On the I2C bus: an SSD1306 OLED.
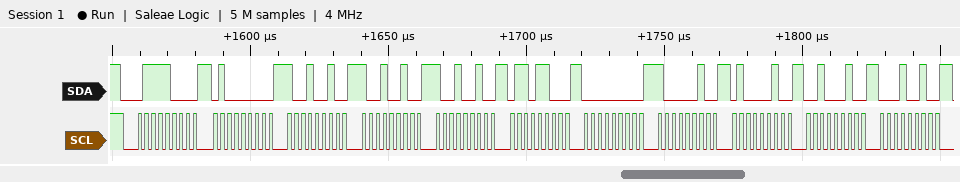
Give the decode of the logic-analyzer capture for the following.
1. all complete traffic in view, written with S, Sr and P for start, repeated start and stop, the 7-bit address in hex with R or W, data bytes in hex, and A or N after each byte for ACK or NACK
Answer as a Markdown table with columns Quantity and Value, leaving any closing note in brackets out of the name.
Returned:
| Quantity | Value |
|---|---|
| all complete traffic in view, written with S, Sr and P for start, repeated start and stop, the 7-bit address in hex with R or W, data bytes in hex, and A or N after each byte for ACK or NACK | S 3CW A 40 A 92 A 92 A 92 A 6C A 00 A 82 A 42 A 22 A 12 A |
